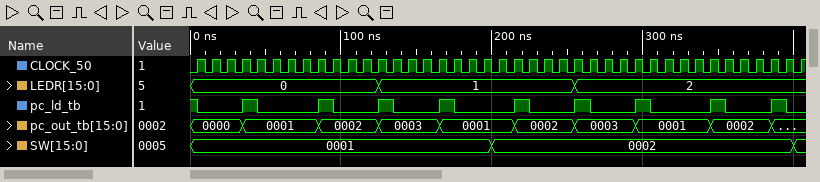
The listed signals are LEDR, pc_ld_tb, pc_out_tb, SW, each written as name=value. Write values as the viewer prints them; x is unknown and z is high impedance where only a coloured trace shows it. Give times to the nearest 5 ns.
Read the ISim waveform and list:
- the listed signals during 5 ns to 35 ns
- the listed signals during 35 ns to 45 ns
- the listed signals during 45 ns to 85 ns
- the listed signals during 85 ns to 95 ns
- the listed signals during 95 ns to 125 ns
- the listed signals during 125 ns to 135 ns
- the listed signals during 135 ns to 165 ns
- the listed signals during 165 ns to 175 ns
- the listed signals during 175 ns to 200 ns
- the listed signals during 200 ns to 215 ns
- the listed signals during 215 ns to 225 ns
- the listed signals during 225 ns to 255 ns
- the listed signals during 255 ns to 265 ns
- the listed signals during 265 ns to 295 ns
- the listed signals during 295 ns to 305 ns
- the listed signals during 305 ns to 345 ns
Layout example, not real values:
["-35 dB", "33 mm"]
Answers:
["LEDR=0, pc_ld_tb=0, pc_out_tb=0000, SW=0001", "LEDR=0, pc_ld_tb=1, pc_out_tb=0001, SW=0001", "LEDR=0, pc_ld_tb=0, pc_out_tb=0001, SW=0001", "LEDR=0, pc_ld_tb=1, pc_out_tb=0002, SW=0001", "LEDR=0, pc_ld_tb=0, pc_out_tb=0002, SW=0001", "LEDR=1, pc_ld_tb=1, pc_out_tb=0003, SW=0001", "LEDR=1, pc_ld_tb=0, pc_out_tb=0003, SW=0001", "LEDR=1, pc_ld_tb=1, pc_out_tb=0001, SW=0001", "LEDR=1, pc_ld_tb=0, pc_out_tb=0001, SW=0001", "LEDR=1, pc_ld_tb=0, pc_out_tb=0001, SW=0002", "LEDR=1, pc_ld_tb=1, pc_out_tb=0002, SW=0002", "LEDR=1, pc_ld_tb=0, pc_out_tb=0002, SW=0002", "LEDR=2, pc_ld_tb=1, pc_out_tb=0003, SW=0002", "LEDR=2, pc_ld_tb=0, pc_out_tb=0003, SW=0002", "LEDR=2, pc_ld_tb=1, pc_out_tb=0001, SW=0002", "LEDR=2, pc_ld_tb=0, pc_out_tb=0001, SW=0002"]
